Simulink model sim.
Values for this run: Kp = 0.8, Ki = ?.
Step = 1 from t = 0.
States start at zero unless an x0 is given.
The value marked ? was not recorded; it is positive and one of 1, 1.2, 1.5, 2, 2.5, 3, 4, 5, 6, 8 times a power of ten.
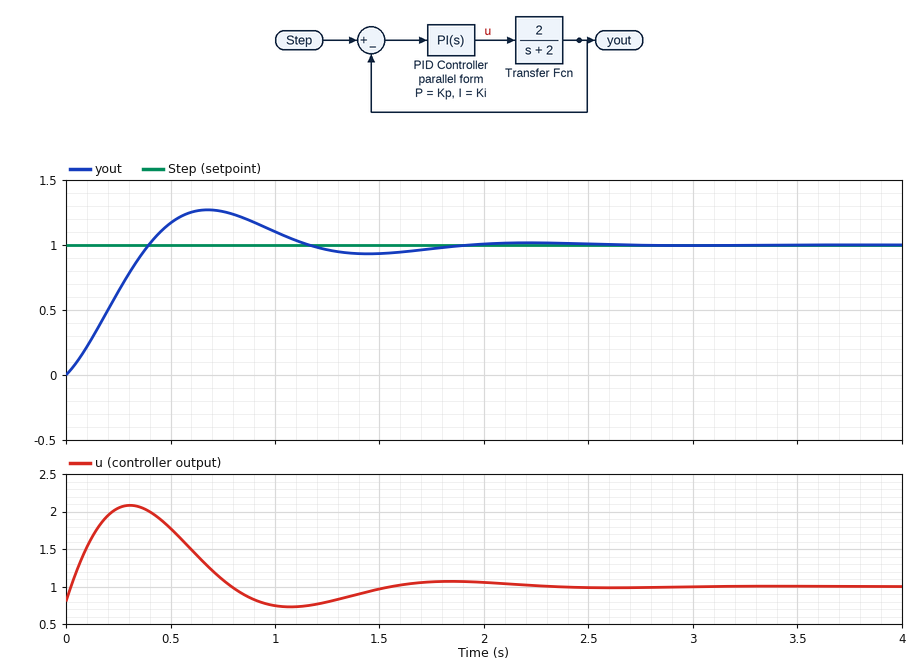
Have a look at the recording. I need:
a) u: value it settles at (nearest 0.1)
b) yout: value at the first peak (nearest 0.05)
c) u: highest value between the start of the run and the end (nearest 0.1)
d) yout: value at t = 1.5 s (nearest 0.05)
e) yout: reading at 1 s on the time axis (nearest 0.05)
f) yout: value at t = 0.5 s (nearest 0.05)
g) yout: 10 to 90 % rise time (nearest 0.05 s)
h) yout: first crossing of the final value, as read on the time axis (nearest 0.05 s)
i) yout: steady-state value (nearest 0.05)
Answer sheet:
1.0
1.25
2.1
0.95
1.10
1.15
0.30 s
0.40 s
1.00
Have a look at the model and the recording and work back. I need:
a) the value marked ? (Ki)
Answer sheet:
10
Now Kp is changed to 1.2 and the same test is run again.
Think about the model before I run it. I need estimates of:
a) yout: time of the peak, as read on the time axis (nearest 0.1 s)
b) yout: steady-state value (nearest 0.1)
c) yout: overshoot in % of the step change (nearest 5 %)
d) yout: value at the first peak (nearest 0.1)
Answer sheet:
0.7 s
1.0
20 %
1.2
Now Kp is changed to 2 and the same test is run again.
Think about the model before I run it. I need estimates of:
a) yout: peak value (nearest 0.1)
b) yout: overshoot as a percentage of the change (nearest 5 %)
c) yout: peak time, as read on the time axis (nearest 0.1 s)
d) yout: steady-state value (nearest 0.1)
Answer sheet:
1.1
10 %
0.6 s
1.0
